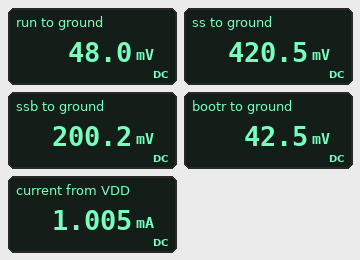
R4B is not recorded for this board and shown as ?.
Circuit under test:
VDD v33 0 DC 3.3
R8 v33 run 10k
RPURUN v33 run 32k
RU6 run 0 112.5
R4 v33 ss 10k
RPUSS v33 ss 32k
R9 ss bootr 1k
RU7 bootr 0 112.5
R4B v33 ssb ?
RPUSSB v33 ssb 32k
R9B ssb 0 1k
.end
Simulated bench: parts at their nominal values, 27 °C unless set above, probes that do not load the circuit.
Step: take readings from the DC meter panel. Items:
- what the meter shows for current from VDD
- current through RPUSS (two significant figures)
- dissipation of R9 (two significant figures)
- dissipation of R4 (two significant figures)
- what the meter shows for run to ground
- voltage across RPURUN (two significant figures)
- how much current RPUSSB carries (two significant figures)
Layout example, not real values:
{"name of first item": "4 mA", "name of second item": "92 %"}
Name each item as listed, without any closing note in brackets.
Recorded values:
{"what the meter shows for current from VDD": "1.005 mA", "current through RPUSS": "90 µA", "dissipation of R9": "140 µW", "dissipation of R4": "830 µW", "what the meter shows for run to ground": "48.0 mV", "voltage across RPURUN": "3.3 V", "how much current RPUSSB carries": "97 µA"}
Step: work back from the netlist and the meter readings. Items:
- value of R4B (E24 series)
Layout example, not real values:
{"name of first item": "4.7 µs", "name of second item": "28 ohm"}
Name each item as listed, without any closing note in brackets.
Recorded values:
{"value of R4B": "30 kΩ"}
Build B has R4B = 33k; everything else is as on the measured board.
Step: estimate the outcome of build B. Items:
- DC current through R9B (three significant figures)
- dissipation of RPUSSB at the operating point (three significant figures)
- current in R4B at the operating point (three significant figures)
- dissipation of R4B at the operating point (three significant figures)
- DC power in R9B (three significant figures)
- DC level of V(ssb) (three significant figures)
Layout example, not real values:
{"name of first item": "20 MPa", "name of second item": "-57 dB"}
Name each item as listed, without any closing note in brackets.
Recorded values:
{"DC current through R9B": "191 µA", "dissipation of RPUSSB at the operating point": "302 µW", "current in R4B at the operating point": "94.2 µA", "dissipation of R4B at the operating point": "293 µW", "DC power in R9B": "36.6 µW", "DC level of V(ssb)": "191 mV"}
